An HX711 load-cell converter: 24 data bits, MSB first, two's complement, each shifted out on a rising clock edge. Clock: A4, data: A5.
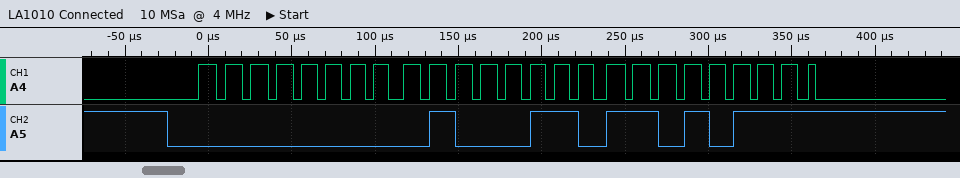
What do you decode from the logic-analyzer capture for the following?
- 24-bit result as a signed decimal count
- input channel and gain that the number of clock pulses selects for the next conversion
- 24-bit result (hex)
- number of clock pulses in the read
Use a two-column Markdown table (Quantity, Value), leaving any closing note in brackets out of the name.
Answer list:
| Quantity | Value |
|---|---|
| 24-bit result as a signed decimal count | 18135 |
| input channel and gain that the number of clock pulses selects for the next conversion | channel A, gain 128 |
| 24-bit result | 0x0046D7 |
| number of clock pulses in the read | 25 |
